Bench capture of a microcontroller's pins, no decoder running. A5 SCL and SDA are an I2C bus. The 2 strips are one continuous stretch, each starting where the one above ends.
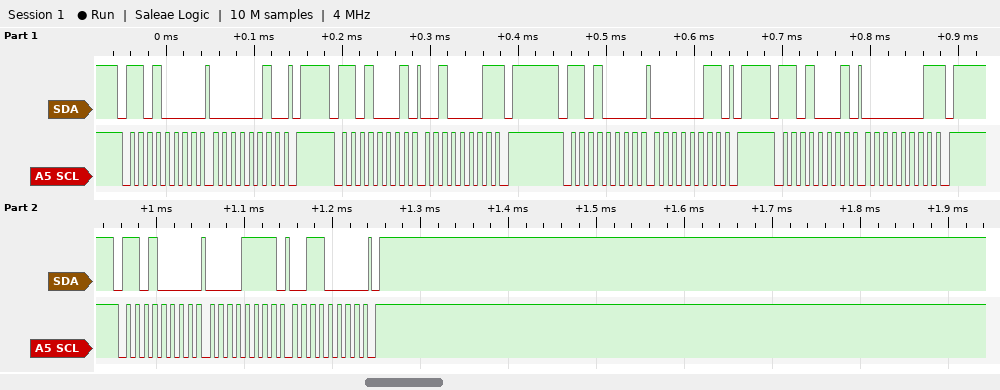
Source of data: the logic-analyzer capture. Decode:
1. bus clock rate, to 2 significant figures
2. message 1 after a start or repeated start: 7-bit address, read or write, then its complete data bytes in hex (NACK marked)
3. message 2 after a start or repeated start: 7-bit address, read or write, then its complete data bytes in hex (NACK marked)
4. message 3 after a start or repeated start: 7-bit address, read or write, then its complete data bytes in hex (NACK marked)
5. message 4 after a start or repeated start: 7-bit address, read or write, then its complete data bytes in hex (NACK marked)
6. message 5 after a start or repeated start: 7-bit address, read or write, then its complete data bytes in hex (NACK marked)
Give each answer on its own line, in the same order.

100 kHz
0x68 write: 02
0x68 read: 21 NACK
0x68 write: 03
0x68 read: 01 NACK
0x68 write: 0F 30
